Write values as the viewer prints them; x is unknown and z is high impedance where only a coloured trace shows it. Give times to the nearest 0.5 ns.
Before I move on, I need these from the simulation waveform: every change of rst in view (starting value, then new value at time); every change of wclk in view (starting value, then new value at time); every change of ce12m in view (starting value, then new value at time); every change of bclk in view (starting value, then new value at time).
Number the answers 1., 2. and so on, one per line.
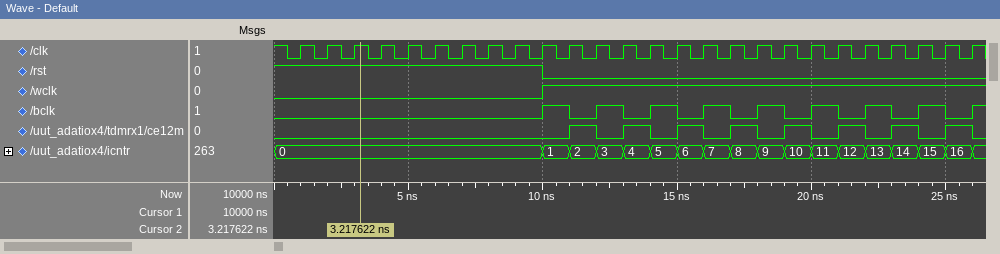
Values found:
1. 1, 0 at 10 ns
2. 0, 1 at 10 ns
3. 0, 1 at 11 ns, 0 at 12 ns, 1 at 13 ns, 0 at 14 ns, 1 at 15 ns, 0 at 16 ns, 1 at 17 ns, 0 at 18 ns, 1 at 19 ns, 0 at 20 ns, 1 at 21 ns, 0 at 22 ns, 1 at 23 ns, 0 at 24 ns, 1 at 25 ns, 0 at 26 ns
4. 0, 1 at 10 ns, 0 at 11 ns, 1 at 12 ns, 0 at 13 ns, 1 at 14 ns, 0 at 15 ns, 1 at 16 ns, 0 at 17 ns, 1 at 18 ns, 0 at 19 ns, 1 at 20 ns, 0 at 21 ns, 1 at 22 ns, 0 at 23 ns, 1 at 24 ns, 0 at 25 ns, 1 at 26 ns
